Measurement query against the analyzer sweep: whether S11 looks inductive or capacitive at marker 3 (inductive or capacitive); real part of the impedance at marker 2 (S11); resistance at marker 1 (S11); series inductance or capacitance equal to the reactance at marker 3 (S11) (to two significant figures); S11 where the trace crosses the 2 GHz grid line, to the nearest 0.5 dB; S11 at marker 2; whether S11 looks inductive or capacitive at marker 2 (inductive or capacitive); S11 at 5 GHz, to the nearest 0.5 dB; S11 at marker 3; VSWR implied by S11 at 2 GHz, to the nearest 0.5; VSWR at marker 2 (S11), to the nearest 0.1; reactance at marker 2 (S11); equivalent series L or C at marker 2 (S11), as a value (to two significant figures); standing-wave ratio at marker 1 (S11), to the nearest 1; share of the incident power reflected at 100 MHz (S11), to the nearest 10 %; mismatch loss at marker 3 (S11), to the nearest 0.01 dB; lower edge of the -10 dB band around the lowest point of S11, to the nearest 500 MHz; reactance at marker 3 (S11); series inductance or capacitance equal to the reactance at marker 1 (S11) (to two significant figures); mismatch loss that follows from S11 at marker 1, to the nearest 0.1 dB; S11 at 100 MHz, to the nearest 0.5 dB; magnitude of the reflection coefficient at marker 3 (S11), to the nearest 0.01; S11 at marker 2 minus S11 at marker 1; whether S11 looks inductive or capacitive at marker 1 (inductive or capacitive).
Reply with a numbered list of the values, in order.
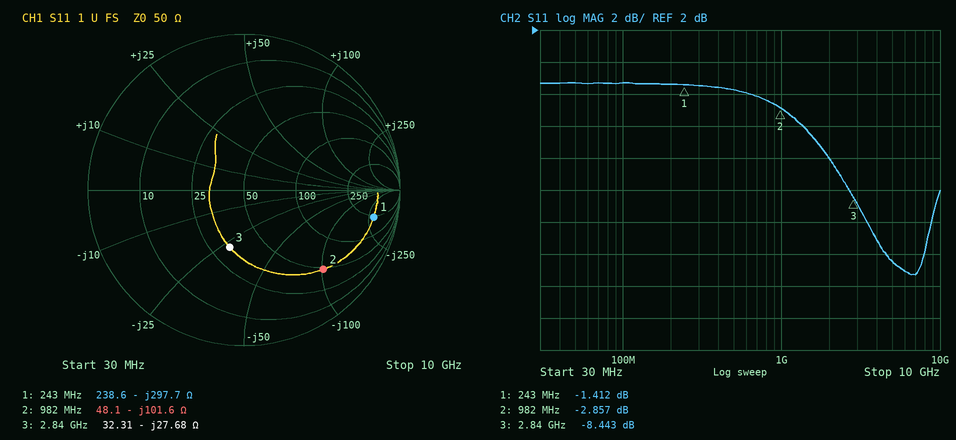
1. capacitive
2. 48.1 Ω
3. 238.6 Ω
4. 2.0 pF
5. -6.0 dB
6. -2.857 dB
7. capacitive
8. -12.5 dB
9. -8.443 dB
10. 3.0
11. 6.1
12. -101.6 Ω
13. 1.6 pF
14. 12
15. 70 %
16. 0.67 dB
17. 3.5 GHz
18. -27.68 Ω
19. 2.2 pF
20. 5.6 dB
21. -1.5 dB
22. 0.38
23. -1.445 dB
24. capacitive
